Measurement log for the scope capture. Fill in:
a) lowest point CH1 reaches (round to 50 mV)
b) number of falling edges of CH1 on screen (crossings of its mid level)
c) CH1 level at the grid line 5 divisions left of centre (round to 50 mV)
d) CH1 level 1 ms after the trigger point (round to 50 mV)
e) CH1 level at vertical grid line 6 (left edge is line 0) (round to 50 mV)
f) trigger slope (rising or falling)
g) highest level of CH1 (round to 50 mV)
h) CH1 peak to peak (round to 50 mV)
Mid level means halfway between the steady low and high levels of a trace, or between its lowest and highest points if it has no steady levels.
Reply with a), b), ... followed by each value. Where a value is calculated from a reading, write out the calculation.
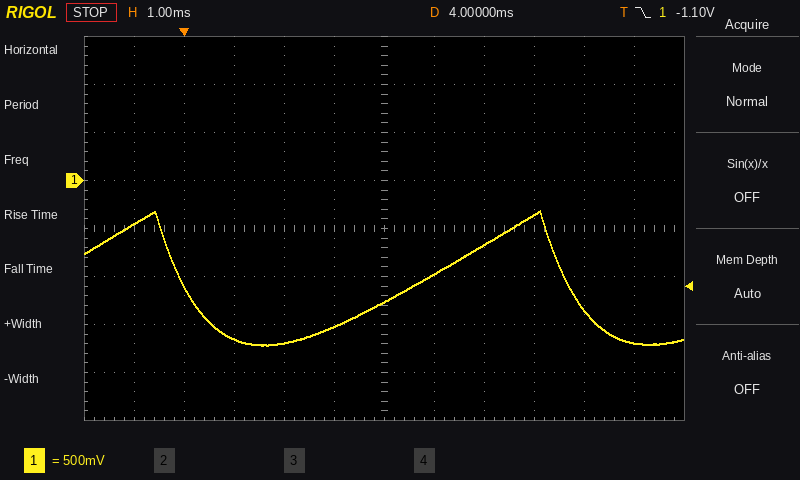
a) -1.70 V
b) 2
c) -450 mV
d) -1.65 V
e) -1.25 V
f) falling
g) -300 mV
h) -300 mV − (-1.70 V) = 1.40 V
